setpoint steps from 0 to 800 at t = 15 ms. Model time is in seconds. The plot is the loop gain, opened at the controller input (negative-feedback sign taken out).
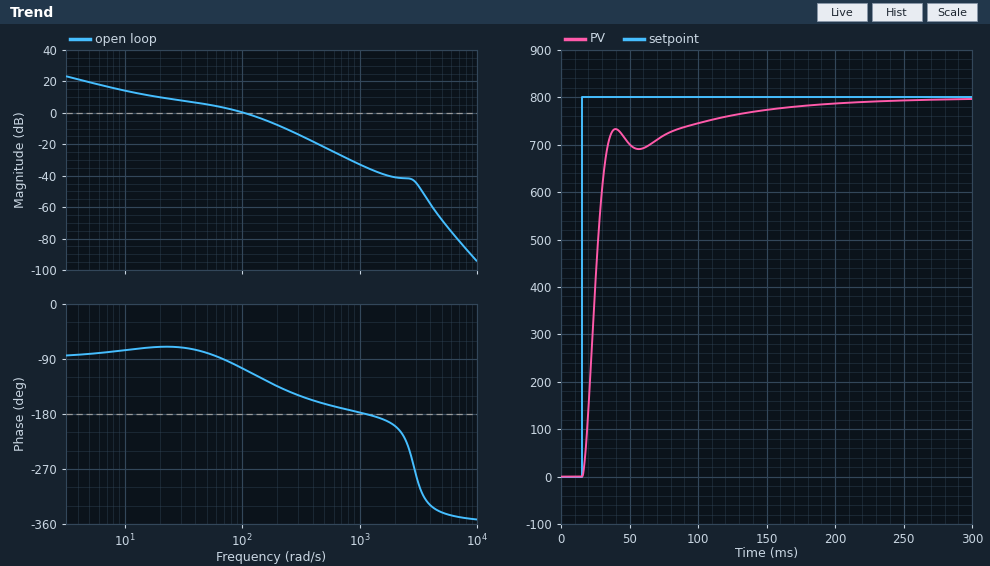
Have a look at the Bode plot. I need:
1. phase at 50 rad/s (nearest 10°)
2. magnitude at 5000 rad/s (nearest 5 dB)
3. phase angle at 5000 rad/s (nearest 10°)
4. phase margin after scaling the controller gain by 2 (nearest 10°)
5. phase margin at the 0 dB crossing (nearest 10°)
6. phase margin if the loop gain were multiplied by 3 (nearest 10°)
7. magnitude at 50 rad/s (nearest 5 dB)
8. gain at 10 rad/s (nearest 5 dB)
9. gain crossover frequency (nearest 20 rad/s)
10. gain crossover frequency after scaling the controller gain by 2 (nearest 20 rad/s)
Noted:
-80°
-70 dB
-340°
50°
70°
40°
5 dB
15 dB
100 rad/s
180 rad/s
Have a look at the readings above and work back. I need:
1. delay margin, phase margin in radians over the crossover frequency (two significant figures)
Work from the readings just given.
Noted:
0.012 s
